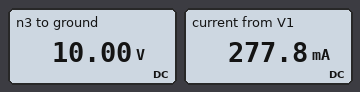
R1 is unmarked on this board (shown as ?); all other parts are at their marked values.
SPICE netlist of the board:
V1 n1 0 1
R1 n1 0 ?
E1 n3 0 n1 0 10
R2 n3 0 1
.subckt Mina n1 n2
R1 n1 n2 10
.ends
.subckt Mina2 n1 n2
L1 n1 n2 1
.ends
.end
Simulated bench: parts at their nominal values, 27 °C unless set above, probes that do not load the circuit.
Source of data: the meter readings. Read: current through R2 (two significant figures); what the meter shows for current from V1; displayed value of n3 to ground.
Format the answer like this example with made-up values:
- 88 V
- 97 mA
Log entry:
- 10 A
- 277.8 mA
- 10.00 V
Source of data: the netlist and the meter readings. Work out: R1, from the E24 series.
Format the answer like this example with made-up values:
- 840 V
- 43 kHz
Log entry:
- 3.6 Ω
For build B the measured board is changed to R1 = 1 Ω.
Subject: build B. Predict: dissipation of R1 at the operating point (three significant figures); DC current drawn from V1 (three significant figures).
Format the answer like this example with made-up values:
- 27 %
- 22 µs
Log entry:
- 1.00 W
- 1.00 A
